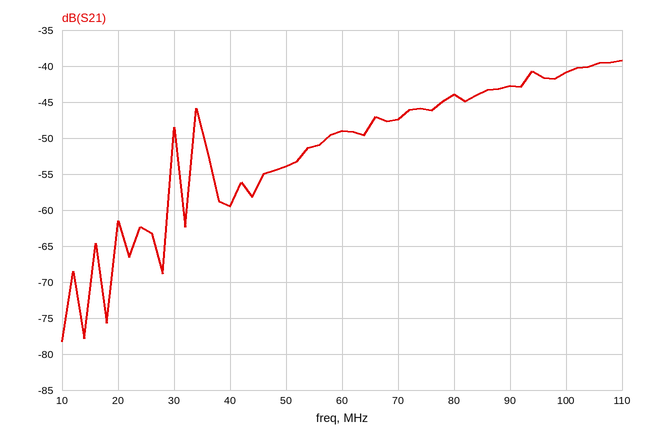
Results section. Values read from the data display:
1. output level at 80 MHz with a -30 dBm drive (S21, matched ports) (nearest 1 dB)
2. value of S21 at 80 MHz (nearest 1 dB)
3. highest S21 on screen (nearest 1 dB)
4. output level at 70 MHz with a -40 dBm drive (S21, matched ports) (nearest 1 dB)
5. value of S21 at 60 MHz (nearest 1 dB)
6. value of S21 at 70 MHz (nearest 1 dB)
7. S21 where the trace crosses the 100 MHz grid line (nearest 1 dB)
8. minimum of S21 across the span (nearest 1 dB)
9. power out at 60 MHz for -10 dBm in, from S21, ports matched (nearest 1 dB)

-74 dBm
-44 dB
-39 dB
-87 dBm
-49 dB
-47 dB
-41 dB
-78 dB
-59 dBm
